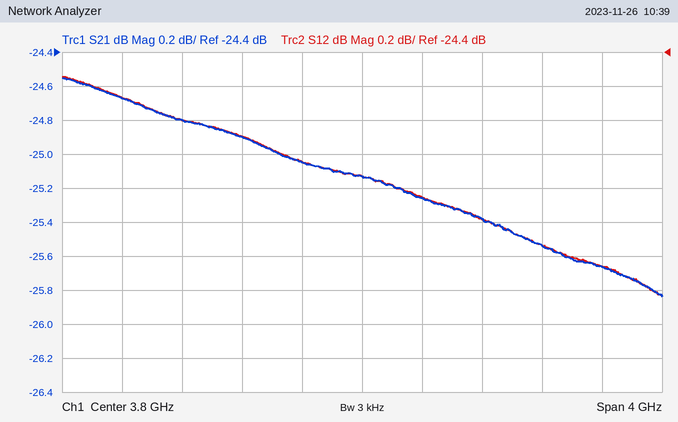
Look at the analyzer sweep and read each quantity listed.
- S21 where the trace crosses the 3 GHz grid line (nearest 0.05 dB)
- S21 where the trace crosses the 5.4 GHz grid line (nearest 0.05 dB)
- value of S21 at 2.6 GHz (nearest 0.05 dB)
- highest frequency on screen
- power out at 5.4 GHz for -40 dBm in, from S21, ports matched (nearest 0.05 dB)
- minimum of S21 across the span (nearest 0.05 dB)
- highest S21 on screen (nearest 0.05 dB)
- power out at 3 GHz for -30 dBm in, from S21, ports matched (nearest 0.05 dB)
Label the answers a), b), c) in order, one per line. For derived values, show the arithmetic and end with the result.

a) -24.90 dB
b) -25.65 dB
c) -24.80 dB
d) 5.8 GHz
e) -40 dBm + (-25.65 dB) = -65.65 dBm
f) -25.85 dB
g) -24.55 dB
h) -30 dBm + (-24.90 dB) = -54.90 dBm
